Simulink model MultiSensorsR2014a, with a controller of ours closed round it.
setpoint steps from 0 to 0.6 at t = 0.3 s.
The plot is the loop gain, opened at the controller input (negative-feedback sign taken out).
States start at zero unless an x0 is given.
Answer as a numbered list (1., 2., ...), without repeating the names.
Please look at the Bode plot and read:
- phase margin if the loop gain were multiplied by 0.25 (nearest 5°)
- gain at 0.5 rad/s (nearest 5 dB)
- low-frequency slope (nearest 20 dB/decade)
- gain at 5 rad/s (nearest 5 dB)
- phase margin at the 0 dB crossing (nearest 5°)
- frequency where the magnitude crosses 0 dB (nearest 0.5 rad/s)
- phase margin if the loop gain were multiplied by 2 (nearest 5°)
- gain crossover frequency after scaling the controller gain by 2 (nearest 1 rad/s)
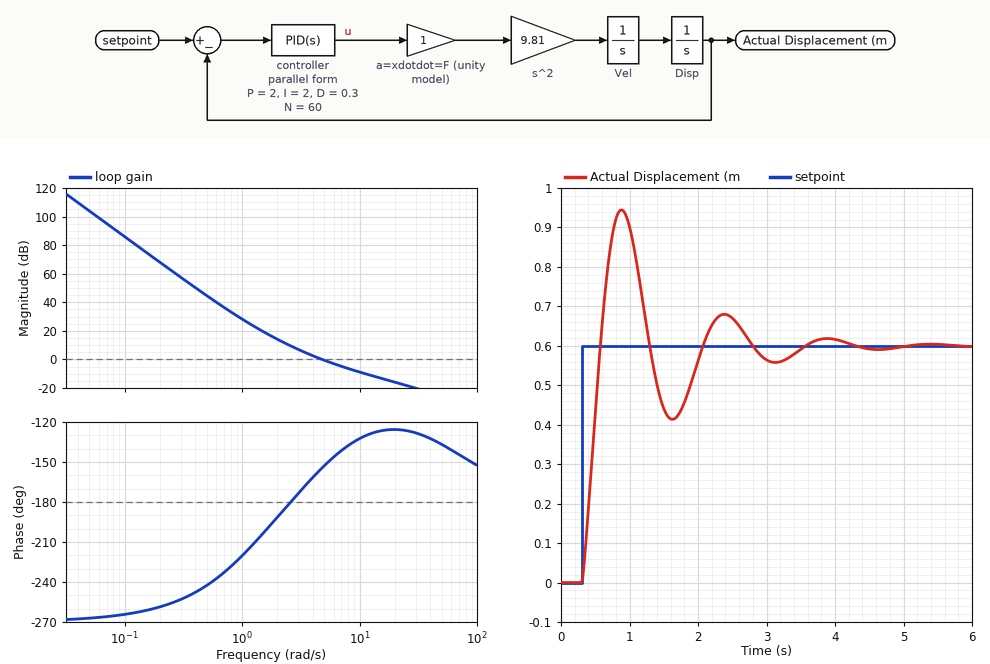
1. -5°
2. 45 dB
3. -60 dB/decade
4. 0 dB
5. 25°
6. 5.0 rad/s
7. 40°
8. 8 rad/s
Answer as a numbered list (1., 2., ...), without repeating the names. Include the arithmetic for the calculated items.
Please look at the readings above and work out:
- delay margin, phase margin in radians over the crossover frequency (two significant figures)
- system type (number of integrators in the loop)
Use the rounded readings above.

1. 25 × π / 180 / 5 = 0.087 s
2. 3
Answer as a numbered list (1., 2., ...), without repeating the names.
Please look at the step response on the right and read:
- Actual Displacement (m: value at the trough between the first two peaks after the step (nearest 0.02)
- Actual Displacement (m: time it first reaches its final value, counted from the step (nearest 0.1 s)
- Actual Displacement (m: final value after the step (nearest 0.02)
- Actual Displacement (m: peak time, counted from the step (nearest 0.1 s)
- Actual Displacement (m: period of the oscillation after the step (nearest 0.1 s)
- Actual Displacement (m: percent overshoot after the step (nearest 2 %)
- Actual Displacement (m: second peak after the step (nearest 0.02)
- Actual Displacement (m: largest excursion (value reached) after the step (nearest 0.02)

1. 0.42
2. 0.3 s
3. 0.60
4. 0.6 s
5. 1.5 s
6. 58 %
7. 0.68
8. 0.94
